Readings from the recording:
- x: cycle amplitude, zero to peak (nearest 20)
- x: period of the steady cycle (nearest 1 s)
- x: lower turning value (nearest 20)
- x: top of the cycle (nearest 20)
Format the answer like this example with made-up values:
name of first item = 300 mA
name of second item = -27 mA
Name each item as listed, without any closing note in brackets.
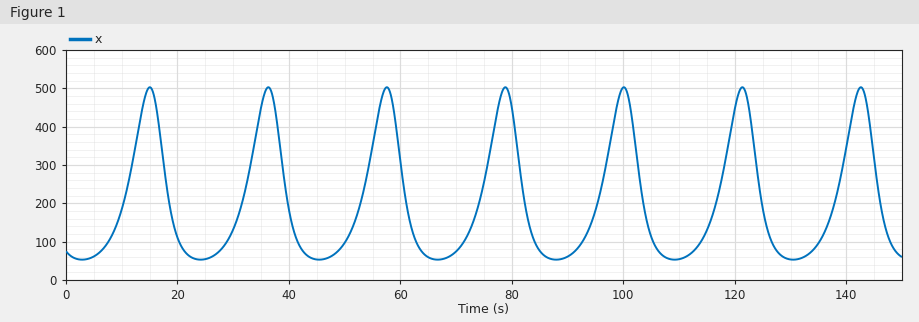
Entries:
x: cycle amplitude, zero to peak = 220
x: period of the steady cycle = 21 s
x: lower turning value = 60
x: top of the cycle = 500
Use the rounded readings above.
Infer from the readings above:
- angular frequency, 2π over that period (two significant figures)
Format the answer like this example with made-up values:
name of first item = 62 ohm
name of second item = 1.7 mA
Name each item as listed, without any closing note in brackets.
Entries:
angular frequency, 2π over that period = 0.30 rad/s
